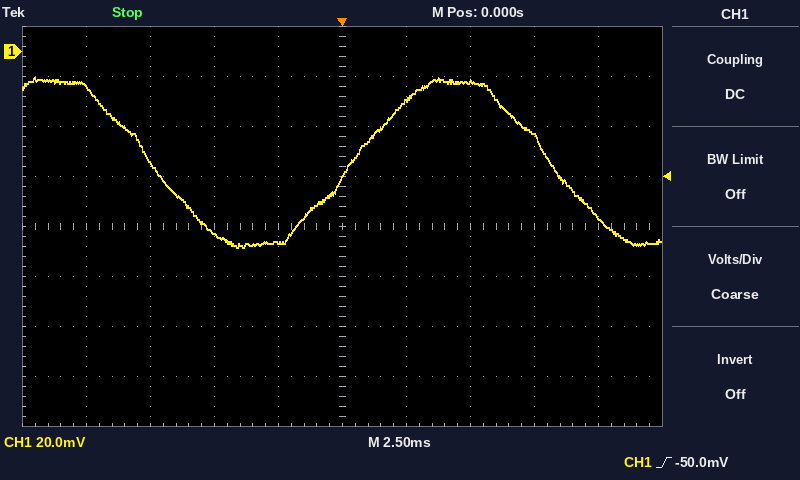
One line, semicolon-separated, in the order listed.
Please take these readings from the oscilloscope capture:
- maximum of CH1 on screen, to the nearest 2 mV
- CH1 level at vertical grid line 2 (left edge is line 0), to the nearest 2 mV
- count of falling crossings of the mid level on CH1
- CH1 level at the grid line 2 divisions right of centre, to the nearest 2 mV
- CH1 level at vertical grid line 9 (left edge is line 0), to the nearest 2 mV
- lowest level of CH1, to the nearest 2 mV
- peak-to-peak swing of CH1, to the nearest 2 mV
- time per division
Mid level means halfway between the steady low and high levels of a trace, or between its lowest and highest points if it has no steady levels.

-10 mV; -44 mV; 2; -12 mV; -66 mV; -78 mV; 68 mV; 2.5 ms
